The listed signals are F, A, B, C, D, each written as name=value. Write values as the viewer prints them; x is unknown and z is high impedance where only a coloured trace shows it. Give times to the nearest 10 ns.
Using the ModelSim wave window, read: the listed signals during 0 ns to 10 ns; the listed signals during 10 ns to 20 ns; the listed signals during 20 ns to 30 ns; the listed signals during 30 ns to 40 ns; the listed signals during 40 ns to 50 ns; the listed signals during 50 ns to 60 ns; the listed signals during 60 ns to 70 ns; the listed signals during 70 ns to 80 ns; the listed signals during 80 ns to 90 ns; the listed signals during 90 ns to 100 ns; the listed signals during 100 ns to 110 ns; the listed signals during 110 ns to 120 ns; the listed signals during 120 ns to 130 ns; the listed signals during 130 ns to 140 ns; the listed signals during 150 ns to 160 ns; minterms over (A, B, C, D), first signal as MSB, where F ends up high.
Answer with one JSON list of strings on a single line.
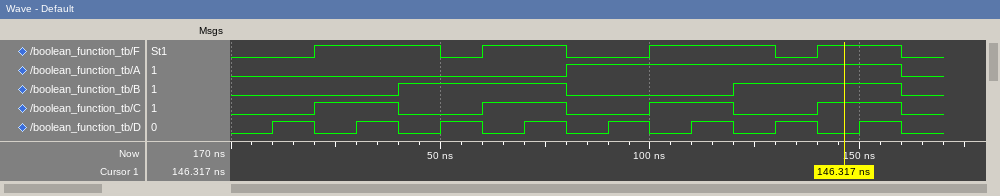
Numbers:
["F=0, A=0, B=0, C=0, D=0", "F=0, A=0, B=0, C=0, D=1", "F=1, A=0, B=0, C=1, D=0", "F=1, A=0, B=0, C=1, D=1", "F=1, A=0, B=1, C=0, D=0", "F=0, A=0, B=1, C=0, D=1", "F=1, A=0, B=1, C=1, D=0", "F=1, A=0, B=1, C=1, D=1", "F=0, A=1, B=0, C=0, D=0", "F=0, A=1, B=0, C=0, D=1", "F=1, A=1, B=0, C=1, D=0", "F=1, A=1, B=0, C=1, D=1", "F=1, A=1, B=1, C=0, D=0", "F=0, A=1, B=1, C=0, D=1", "F=1, A=1, B=1, C=1, D=1", "2, 3, 4, 6, 7, 10, 11, 12, 14, 15"]
